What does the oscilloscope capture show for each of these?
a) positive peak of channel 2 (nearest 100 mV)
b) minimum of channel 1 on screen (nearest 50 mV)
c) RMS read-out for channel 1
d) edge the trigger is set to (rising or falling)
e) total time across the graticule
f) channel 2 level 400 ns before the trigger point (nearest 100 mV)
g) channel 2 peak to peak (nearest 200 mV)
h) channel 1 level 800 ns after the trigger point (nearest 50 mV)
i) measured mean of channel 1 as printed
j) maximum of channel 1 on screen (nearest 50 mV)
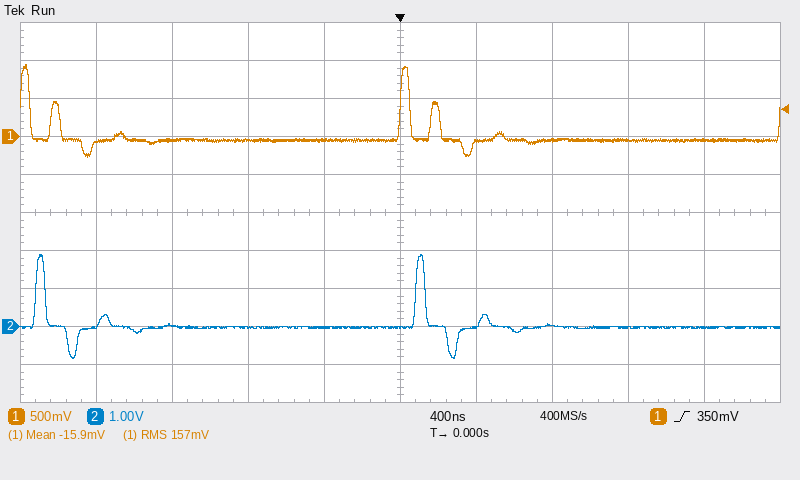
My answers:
1.9 V
-300 mV
157 mV
rising
4 µs
0.0 V
2.8 V
-50 mV
-15.9 mV
950 mV
